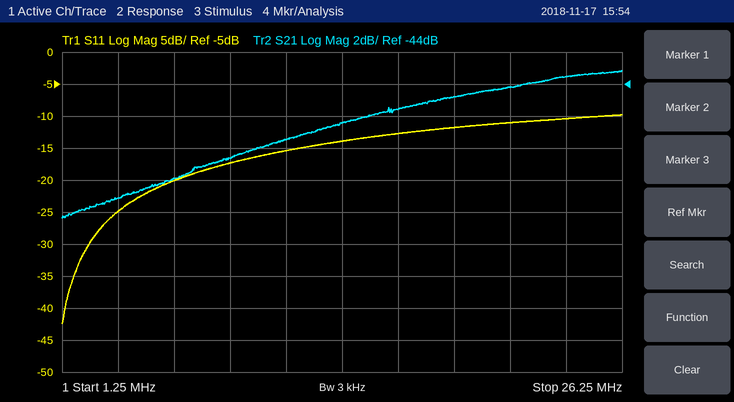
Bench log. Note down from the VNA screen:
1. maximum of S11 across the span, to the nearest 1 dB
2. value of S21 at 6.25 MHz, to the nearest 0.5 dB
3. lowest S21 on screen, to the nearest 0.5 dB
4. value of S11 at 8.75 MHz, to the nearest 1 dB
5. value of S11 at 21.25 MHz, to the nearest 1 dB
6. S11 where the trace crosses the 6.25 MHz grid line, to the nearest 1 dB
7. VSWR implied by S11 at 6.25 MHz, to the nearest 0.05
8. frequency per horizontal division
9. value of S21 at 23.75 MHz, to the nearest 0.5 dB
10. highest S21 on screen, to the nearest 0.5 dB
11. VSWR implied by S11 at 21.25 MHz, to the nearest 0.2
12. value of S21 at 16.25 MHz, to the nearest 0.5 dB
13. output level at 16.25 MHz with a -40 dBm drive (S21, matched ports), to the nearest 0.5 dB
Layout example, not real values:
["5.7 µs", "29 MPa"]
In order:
["-10 dB", "-50.0 dB", "-52.5 dB", "-17 dB", "-11 dB", "-20 dB", "1.20", "2.5 MHz", "-43.5 dB", "-43.0 dB", "1.8", "-45.5 dB", "-85.5 dBm"]
